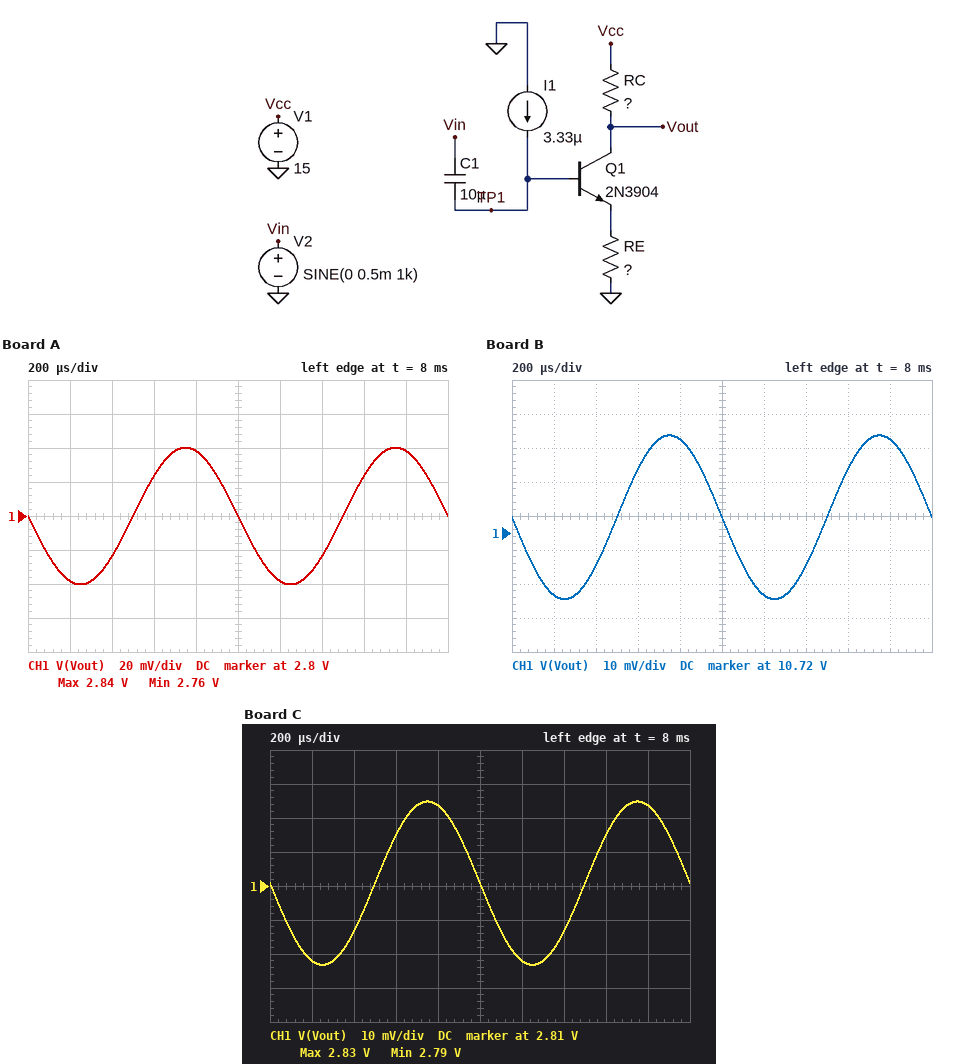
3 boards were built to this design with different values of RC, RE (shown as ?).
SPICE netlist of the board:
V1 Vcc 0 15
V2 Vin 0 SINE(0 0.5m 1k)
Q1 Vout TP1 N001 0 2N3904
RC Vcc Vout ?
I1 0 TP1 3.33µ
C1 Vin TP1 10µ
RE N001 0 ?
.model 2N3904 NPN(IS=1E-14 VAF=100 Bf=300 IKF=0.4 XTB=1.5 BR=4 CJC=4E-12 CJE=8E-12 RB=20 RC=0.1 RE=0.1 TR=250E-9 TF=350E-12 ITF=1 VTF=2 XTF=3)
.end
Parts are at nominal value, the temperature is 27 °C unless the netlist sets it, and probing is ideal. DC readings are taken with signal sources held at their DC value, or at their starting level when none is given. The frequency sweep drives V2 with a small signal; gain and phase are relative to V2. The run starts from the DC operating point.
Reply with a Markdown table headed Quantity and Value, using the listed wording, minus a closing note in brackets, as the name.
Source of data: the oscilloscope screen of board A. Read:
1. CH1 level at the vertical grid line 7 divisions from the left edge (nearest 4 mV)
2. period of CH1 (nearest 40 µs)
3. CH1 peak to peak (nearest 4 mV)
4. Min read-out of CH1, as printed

| Quantity | Value |
|---|---|
| CH1 level at the vertical grid line 7 divisions from the left edge | 2.776 V |
| period of CH1 | 1.00 ms |
| CH1 peak to peak | 80 mV |
| Min read-out of CH1, as printed | 2.76 V |
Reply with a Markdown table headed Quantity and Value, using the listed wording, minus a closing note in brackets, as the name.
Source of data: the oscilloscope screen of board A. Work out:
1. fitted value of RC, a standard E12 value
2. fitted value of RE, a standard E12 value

| Quantity | Value |
|---|---|
| fitted value of RC, a standard E12 value | 12 kΩ |
| fitted value of RE, a standard E12 value | 120 Ω |
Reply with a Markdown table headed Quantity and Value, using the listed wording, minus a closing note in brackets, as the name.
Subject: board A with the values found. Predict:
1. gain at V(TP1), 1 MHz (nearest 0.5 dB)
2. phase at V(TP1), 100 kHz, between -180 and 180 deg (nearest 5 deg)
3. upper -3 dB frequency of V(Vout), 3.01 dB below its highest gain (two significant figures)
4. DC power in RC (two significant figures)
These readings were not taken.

| Quantity | Value |
|---|---|
| gain at V(TP1), 1 MHz | 0 dB |
| phase at V(TP1), 100 kHz, between -180 and 180 deg | 0 deg |
| upper -3 dB frequency of V(Vout), 3.01 dB below its highest gain | 4.6 MHz |
| DC power in RC | 12 mW |
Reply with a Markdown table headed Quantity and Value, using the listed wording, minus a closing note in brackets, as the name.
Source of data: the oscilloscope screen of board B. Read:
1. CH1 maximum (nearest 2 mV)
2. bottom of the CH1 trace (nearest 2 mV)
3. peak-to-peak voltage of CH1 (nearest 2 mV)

| Quantity | Value |
|---|---|
| CH1 maximum | 10.748 V |
| bottom of the CH1 trace | 10.700 V |
| peak-to-peak voltage of CH1 | 48 mV |
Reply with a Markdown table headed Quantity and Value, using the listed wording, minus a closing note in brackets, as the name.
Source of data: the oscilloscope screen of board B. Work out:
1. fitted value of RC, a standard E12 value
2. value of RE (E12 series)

| Quantity | Value |
|---|---|
| fitted value of RC, a standard E12 value | 3.9 kΩ |
| value of RE | 56 Ω |
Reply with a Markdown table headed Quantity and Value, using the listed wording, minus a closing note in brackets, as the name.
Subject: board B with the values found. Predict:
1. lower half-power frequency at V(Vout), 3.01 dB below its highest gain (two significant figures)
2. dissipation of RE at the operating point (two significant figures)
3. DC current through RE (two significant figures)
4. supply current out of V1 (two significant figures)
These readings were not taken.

| Quantity | Value |
|---|---|
| lower half-power frequency at V(Vout), 3.01 dB below its highest gain | 620 mHz |
| dissipation of RE at the operating point | 68 µW |
| DC current through RE | 1.1 mA |
| supply current out of V1 | 1.1 mA |
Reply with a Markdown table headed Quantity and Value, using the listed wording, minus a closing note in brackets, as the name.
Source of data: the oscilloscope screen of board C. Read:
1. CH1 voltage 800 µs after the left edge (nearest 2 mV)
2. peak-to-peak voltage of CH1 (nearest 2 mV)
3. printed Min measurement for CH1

| Quantity | Value |
|---|---|
| CH1 voltage 800 µs after the left edge | 2.834 V |
| peak-to-peak voltage of CH1 | 48 mV |
| printed Min measurement for CH1 | 2.79 V |
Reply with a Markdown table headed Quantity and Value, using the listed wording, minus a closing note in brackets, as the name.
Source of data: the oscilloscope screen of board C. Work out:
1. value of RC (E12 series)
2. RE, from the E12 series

| Quantity | Value |
|---|---|
| value of RC | 12 kΩ |
| RE, from the E12 series | 220 Ω |
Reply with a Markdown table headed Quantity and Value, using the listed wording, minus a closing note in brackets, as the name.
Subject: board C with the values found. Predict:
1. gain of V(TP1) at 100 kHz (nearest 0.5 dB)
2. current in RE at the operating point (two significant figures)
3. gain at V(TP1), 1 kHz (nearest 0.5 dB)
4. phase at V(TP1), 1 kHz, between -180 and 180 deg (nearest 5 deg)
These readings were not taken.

| Quantity | Value |
|---|---|
| gain of V(TP1) at 100 kHz | 0 dB |
| current in RE at the operating point | 1.0 mA |
| gain at V(TP1), 1 kHz | 0 dB |
| phase at V(TP1), 1 kHz, between -180 and 180 deg | 0 deg |
